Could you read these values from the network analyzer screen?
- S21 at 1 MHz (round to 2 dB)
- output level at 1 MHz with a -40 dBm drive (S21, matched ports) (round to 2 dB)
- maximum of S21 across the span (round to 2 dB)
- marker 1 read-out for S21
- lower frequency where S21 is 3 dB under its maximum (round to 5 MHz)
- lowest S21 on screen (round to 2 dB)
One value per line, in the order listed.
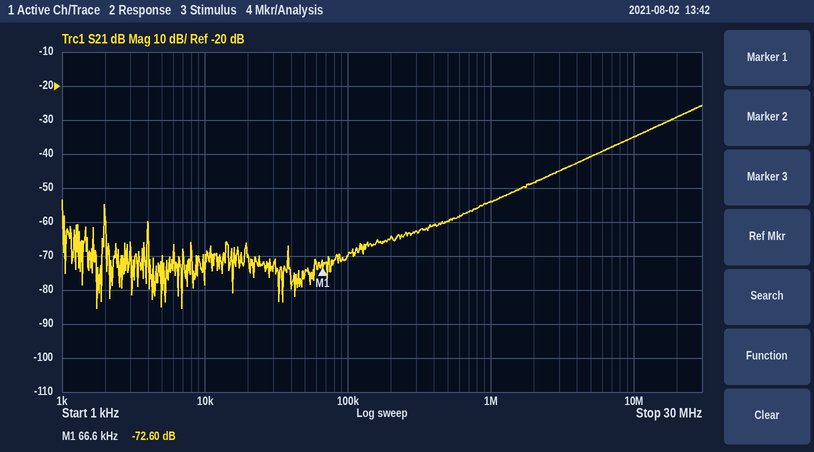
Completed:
-54 dB
-94 dBm
-26 dB
-72.60 dB
20 MHz
-86 dB
